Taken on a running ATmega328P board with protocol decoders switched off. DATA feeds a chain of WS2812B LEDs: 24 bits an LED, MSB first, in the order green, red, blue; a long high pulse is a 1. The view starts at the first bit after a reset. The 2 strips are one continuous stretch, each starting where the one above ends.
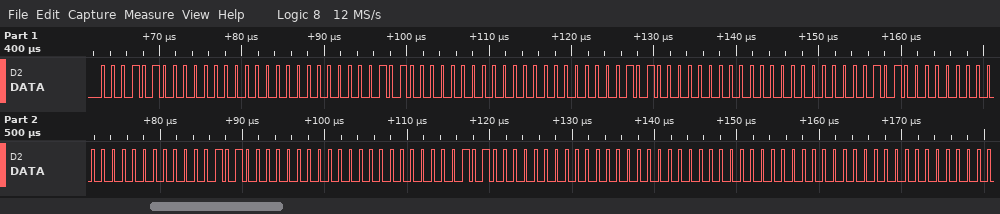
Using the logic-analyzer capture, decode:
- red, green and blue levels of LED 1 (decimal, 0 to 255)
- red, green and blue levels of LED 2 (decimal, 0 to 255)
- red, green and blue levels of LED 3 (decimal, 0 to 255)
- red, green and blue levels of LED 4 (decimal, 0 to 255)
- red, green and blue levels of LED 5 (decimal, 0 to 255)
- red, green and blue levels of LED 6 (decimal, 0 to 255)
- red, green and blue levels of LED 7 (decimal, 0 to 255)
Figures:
0, 20, 0
0, 20, 0
0, 20, 0
0, 20, 0
0, 20, 0
0, 20, 0
0, 0, 0
